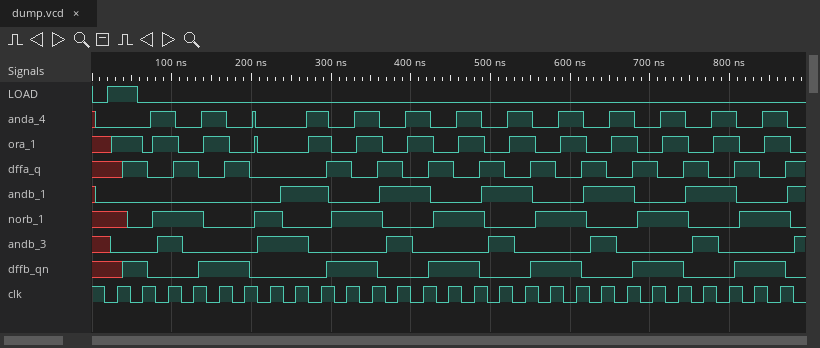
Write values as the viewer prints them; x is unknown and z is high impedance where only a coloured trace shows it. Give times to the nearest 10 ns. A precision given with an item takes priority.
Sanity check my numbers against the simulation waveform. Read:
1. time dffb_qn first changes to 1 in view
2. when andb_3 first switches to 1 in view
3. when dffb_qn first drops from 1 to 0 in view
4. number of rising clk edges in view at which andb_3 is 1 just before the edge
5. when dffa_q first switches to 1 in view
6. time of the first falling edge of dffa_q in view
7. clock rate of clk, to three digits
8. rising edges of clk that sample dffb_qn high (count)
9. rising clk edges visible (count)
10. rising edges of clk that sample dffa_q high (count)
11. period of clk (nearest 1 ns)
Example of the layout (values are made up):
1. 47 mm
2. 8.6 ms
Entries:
1. 40 ns
2. 80 ns
3. 70 ns
4. 7
5. 40 ns
6. 70 ns
7. 31.2 MHz
8. 13
9. 27
10. 12
11. 32 ns
